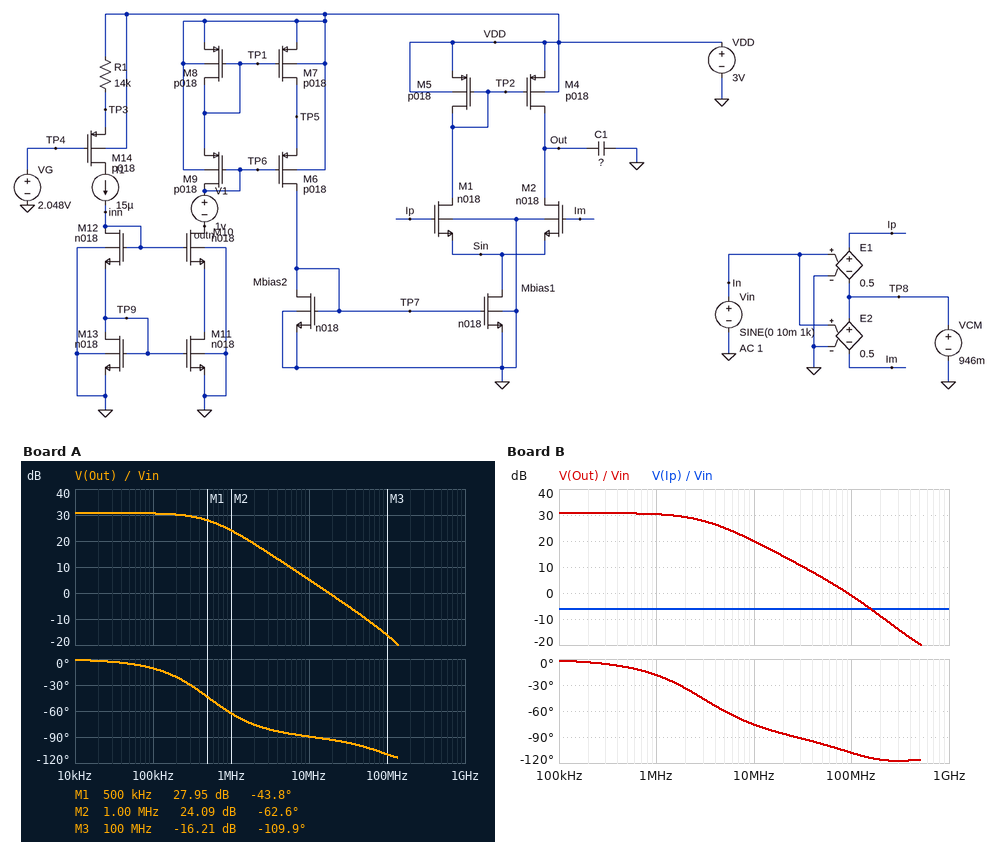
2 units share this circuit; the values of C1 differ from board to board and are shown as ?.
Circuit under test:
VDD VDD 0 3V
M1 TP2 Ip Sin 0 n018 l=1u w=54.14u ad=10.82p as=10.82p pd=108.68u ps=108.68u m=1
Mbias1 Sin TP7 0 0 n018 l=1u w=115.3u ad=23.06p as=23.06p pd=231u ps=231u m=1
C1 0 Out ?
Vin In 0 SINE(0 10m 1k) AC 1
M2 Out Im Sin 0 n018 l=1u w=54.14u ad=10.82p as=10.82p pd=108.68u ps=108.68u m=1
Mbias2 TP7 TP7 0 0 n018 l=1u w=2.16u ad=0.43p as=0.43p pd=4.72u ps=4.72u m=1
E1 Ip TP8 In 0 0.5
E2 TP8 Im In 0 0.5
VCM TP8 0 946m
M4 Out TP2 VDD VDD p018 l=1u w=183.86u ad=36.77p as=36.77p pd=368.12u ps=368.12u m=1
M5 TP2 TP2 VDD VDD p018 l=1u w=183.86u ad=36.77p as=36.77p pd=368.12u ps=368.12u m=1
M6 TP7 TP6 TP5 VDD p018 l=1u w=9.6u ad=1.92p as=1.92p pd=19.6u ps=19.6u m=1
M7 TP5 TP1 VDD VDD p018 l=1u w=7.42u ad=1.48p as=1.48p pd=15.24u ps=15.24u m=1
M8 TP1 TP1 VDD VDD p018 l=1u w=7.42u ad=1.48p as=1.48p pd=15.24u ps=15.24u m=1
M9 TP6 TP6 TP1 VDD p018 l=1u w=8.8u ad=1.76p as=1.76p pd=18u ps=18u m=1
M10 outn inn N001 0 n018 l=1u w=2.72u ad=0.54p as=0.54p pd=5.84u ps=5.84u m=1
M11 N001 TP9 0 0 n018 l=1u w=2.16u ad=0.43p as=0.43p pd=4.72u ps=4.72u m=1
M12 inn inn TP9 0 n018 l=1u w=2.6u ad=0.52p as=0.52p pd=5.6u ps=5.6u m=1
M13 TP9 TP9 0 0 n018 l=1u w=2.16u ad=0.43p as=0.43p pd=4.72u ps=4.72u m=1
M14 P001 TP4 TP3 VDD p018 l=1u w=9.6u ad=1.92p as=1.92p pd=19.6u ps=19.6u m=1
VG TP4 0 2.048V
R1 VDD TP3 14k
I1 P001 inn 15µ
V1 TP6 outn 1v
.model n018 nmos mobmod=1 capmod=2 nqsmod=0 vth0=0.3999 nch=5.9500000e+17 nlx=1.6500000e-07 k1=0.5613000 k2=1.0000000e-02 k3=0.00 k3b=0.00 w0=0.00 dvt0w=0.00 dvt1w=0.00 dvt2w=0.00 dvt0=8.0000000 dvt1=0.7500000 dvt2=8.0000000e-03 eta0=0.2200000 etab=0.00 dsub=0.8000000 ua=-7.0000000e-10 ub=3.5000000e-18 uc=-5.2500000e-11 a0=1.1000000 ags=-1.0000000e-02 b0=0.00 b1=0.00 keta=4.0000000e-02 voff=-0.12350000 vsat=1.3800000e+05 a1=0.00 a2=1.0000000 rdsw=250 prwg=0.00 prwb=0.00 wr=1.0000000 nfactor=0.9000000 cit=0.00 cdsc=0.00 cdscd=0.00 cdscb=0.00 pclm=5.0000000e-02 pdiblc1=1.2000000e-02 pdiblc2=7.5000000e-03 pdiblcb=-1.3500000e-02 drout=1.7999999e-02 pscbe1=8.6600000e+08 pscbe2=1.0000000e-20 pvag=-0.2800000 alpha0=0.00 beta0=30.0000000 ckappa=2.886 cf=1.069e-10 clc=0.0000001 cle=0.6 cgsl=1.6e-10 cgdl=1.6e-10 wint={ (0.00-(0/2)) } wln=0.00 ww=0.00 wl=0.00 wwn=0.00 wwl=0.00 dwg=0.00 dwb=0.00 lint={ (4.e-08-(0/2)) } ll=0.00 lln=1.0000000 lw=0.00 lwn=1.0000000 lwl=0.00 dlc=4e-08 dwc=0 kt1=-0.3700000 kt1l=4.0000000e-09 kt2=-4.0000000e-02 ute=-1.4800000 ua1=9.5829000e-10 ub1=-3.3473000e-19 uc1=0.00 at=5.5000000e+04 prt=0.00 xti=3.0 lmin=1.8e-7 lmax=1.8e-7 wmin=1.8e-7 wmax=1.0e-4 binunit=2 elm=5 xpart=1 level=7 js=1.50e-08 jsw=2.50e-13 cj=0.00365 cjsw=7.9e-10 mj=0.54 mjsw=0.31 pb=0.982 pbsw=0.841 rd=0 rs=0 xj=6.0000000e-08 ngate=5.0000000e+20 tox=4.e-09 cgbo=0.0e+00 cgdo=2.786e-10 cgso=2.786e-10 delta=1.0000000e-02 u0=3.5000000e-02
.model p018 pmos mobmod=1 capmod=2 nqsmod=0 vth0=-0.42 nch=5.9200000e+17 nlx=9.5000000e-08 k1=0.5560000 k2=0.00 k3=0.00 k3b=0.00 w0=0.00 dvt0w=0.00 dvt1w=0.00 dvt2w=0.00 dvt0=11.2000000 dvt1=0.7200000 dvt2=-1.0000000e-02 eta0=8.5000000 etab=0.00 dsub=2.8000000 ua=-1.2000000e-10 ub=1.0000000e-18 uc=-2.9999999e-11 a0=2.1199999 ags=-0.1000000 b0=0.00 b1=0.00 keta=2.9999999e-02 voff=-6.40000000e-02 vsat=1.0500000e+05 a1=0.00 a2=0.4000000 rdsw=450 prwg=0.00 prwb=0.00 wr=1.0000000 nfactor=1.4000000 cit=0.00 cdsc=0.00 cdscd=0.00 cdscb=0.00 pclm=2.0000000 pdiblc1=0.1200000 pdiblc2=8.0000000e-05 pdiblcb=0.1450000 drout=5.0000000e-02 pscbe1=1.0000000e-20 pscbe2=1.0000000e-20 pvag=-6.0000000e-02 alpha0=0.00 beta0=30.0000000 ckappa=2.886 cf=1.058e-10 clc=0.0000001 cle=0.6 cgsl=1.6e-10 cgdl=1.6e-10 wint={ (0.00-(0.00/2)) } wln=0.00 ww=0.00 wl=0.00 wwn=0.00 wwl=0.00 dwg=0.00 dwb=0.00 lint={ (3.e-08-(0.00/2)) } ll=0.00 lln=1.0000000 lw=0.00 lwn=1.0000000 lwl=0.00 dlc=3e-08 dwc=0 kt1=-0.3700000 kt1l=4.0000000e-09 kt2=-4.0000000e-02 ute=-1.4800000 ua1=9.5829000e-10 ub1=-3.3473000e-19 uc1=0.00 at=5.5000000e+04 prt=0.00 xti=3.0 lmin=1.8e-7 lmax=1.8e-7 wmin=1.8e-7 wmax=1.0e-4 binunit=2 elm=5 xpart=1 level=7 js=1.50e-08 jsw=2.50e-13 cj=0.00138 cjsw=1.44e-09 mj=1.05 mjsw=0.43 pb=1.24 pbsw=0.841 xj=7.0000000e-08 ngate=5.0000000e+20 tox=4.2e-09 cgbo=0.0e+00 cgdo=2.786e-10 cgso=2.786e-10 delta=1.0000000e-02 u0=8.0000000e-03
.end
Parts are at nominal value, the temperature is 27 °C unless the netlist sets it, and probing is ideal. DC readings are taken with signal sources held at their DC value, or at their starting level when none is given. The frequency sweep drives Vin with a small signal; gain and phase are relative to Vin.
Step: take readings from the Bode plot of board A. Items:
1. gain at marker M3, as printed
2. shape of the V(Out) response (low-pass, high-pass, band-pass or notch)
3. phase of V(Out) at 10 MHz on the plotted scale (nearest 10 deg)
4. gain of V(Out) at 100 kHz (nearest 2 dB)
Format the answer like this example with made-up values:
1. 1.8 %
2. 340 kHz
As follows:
1. -16.21 dB
2. low-pass
3. -90 deg
4. 30 dB
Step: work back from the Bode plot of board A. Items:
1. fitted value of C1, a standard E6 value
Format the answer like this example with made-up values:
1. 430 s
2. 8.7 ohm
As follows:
1. 22 pF
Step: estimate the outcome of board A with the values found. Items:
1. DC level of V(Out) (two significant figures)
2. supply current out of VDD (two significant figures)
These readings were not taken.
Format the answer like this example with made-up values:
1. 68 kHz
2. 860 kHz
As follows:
1. 2.2 V
2. 1.0 mA
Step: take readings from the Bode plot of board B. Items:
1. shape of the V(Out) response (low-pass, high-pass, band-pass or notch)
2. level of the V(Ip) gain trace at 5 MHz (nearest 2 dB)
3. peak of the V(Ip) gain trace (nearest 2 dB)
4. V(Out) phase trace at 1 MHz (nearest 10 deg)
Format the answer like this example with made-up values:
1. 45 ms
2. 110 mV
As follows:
1. low-pass
2. -6 dB
3. -6 dB
4. -20 deg
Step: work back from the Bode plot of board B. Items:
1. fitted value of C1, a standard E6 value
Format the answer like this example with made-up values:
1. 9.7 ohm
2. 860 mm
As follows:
1. 3.3 pF
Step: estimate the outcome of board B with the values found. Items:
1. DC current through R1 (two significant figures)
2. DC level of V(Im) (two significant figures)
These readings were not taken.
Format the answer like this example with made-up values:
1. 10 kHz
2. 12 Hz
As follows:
1. 15 µA
2. 950 mV
